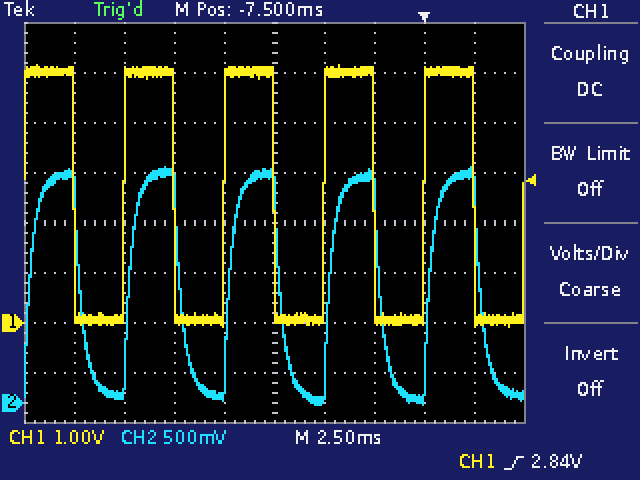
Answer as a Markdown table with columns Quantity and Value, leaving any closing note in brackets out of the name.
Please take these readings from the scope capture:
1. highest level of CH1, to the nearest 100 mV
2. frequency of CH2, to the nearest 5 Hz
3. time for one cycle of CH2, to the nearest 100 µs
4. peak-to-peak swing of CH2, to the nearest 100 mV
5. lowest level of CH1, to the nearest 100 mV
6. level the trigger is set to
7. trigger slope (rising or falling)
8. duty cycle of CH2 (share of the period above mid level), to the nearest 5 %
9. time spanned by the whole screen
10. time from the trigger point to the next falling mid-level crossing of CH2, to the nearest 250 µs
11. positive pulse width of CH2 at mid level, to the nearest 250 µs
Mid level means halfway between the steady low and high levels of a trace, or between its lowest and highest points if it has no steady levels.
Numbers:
| Quantity | Value |
|---|---|
| highest level of CH1, to the nearest 100 mV | 5.2 V |
| frequency of CH2, to the nearest 5 Hz | 200 Hz |
| time for one cycle of CH2, to the nearest 100 µs | 5.0 ms |
| peak-to-peak swing of CH2, to the nearest 100 mV | 2.40 V |
| lowest level of CH1, to the nearest 100 mV | -100 mV |
| level the trigger is set to | 2.84 V |
| trigger slope | rising |
| duty cycle of CH2 (share of the period above mid level), to the nearest 5 % | 50 % |
| time spanned by the whole screen | 25 ms |
| time from the trigger point to the next falling mid-level crossing of CH2, to the nearest 250 µs | 2.75 ms |
| positive pulse width of CH2 at mid level, to the nearest 250 µs | 2.50 ms |
